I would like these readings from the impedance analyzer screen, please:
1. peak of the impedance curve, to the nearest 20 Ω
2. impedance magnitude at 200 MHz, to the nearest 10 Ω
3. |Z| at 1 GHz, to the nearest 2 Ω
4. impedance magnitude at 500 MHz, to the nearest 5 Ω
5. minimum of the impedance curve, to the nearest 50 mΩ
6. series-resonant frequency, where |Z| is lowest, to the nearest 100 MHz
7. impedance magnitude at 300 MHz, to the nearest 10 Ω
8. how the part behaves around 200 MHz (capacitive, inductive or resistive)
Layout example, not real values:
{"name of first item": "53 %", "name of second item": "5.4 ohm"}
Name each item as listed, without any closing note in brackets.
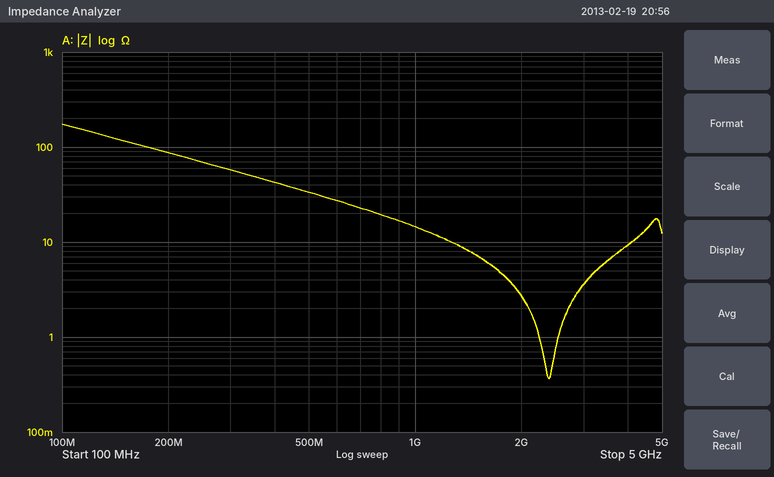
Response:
{"peak of the impedance curve, to the nearest 20 Ω": "180 Ω", "impedance magnitude at 200 MHz, to the nearest 10 Ω": "90 Ω", "|Z| at 1 GHz, to the nearest 2 Ω": "14 Ω", "impedance magnitude at 500 MHz, to the nearest 5 Ω": "35 Ω", "minimum of the impedance curve, to the nearest 50 mΩ": "350 mΩ", "series-resonant frequency, where |Z| is lowest, to the nearest 100 MHz": "2.4 GHz", "impedance magnitude at 300 MHz, to the nearest 10 Ω": "60 Ω", "how the part behaves around 200 MHz": "capacitive"}
